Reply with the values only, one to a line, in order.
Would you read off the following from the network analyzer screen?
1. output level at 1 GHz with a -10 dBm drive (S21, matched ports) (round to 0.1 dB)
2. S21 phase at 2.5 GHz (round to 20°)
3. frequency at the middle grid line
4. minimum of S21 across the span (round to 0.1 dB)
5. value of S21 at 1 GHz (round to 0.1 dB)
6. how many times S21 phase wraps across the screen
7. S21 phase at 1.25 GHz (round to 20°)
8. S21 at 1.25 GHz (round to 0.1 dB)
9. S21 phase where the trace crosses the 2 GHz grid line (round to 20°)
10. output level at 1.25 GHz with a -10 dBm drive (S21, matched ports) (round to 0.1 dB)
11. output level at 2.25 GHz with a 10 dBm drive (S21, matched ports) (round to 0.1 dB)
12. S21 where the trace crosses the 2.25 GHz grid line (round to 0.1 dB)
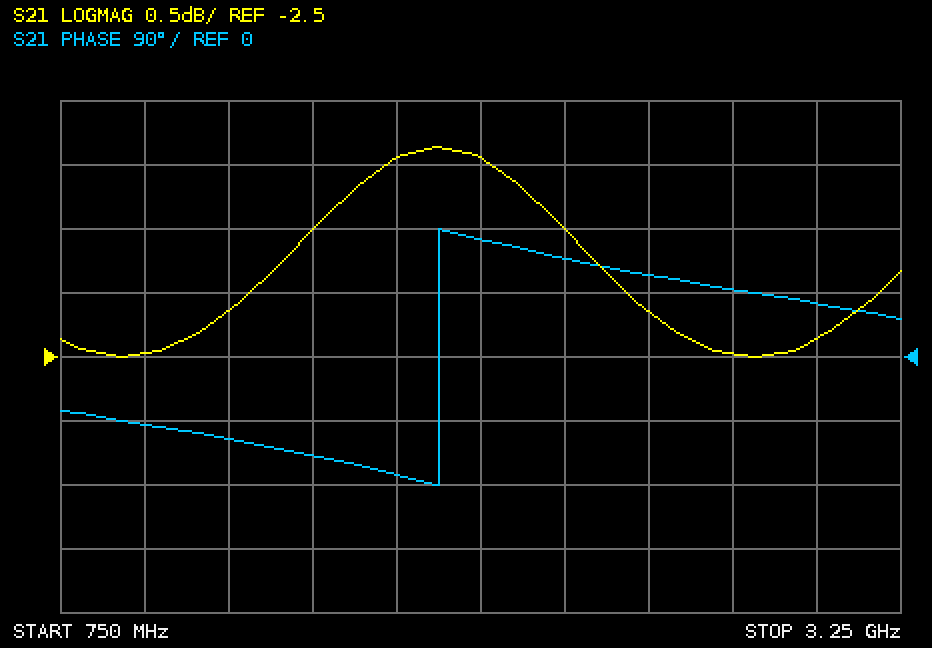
-12.5 dBm
120°
2 GHz
-2.5 dB
-2.5 dB
1
-120°
-2.1 dB
160°
-12.1 dBm
8.5 dBm
-1.5 dB
